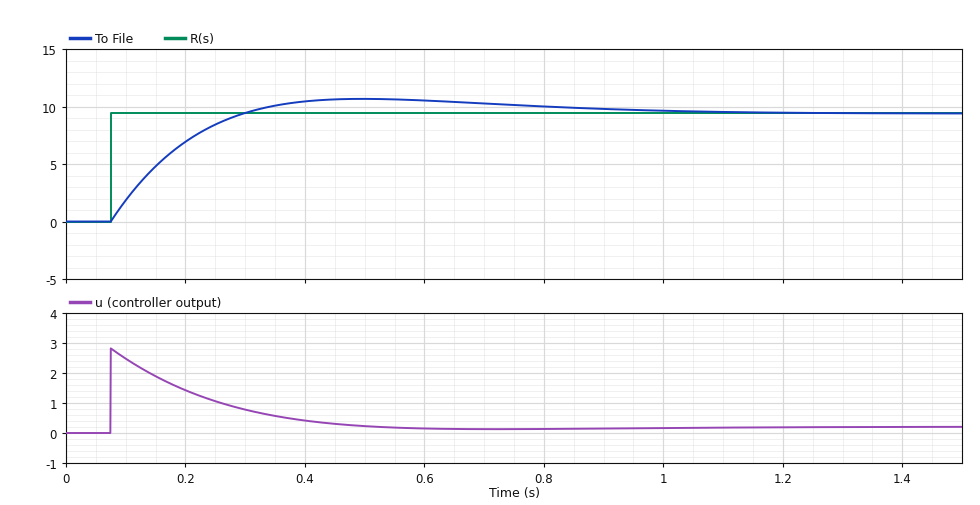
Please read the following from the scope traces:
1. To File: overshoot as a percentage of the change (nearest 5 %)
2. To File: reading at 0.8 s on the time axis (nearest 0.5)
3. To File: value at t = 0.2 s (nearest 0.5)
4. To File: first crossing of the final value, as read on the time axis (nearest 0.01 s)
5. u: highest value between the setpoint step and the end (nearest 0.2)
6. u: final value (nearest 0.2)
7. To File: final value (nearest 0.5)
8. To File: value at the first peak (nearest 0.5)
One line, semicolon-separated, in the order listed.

15 %; 10.0; 7.0; 0.30 s; 2.8; 0.2; 9.5; 10.5
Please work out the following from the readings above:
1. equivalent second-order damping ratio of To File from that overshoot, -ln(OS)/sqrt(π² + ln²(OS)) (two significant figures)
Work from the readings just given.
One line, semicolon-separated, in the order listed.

0.52
